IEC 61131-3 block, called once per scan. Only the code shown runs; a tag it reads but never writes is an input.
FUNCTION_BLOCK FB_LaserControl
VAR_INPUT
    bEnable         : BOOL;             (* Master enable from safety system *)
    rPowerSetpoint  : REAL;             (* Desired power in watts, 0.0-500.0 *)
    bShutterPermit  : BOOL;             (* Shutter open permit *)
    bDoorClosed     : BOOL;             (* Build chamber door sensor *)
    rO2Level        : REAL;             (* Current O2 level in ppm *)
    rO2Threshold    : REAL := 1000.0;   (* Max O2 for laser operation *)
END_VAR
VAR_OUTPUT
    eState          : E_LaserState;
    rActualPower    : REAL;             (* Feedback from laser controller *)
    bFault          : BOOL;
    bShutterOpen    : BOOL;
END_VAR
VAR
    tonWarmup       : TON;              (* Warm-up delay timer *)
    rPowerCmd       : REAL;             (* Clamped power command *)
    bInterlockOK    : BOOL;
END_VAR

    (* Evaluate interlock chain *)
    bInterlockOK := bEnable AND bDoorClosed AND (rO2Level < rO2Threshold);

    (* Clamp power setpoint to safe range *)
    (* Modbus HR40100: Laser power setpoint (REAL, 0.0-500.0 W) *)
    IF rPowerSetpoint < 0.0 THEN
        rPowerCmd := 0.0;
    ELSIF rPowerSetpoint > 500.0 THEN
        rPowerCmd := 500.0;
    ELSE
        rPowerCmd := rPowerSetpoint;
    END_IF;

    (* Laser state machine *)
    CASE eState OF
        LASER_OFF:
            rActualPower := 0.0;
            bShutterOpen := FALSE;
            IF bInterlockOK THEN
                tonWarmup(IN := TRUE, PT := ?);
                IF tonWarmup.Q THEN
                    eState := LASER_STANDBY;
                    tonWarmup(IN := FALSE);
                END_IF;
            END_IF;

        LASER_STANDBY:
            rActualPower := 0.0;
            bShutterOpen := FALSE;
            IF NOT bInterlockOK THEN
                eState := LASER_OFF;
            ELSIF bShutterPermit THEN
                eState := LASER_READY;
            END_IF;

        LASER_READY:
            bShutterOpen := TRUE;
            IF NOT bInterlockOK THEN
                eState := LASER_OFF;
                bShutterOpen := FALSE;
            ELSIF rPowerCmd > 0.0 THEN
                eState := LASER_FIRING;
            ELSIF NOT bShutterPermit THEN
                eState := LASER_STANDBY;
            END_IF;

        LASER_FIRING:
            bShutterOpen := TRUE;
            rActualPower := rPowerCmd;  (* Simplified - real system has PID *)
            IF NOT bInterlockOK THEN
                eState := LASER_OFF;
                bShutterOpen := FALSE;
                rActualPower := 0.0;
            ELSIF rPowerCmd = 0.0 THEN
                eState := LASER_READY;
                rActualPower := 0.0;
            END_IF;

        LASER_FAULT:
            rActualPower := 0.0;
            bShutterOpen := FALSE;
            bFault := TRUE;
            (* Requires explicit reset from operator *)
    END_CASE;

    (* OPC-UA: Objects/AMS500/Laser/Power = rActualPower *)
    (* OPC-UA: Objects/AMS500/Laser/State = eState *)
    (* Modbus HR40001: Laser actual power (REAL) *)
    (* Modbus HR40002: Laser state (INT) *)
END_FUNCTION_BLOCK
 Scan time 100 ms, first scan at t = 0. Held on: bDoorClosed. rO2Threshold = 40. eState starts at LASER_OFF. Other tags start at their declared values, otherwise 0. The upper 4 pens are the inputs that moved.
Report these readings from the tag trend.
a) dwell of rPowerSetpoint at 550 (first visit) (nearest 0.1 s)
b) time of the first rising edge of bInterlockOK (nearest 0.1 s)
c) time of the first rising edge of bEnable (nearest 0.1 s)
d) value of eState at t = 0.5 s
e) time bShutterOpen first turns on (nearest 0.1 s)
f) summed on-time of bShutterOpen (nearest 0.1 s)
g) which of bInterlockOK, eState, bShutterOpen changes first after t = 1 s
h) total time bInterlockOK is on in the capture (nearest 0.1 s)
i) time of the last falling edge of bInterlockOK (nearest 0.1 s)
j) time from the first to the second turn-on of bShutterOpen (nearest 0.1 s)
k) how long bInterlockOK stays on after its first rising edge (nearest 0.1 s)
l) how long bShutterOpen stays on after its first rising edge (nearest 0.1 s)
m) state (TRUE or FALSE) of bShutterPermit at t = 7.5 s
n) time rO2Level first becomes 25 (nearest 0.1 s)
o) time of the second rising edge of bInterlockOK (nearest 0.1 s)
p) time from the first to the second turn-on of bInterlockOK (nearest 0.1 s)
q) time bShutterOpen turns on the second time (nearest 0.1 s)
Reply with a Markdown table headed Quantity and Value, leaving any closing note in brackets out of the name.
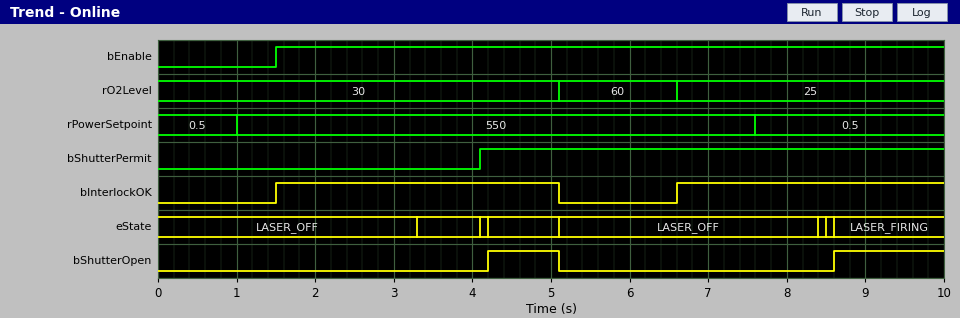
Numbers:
| Quantity | Value |
|---|---|
| dwell of rPowerSetpoint at 550 (first visit) | 6.6 s |
| time of the first rising edge of bInterlockOK | 1.5 s |
| time of the first rising edge of bEnable | 1.5 s |
| value of eState at t = 0.5 s | LASER_OFF |
| time bShutterOpen first turns on | 4.2 s |
| summed on-time of bShutterOpen | 2.3 s |
| which of bInterlockOK, eState, bShutterOpen changes first after t = 1 s | bInterlockOK |
| total time bInterlockOK is on in the capture | 7.0 s |
| time of the last falling edge of bInterlockOK | 5.1 s |
| time from the first to the second turn-on of bShutterOpen | 4.4 s |
| how long bInterlockOK stays on after its first rising edge | 3.6 s |
| how long bShutterOpen stays on after its first rising edge | 0.9 s |
| state (TRUE or FALSE) of bShutterPermit at t = 7.5 s | TRUE |
| time rO2Level first becomes 25 | 6.6 s |
| time of the second rising edge of bInterlockOK | 6.6 s |
| time from the first to the second turn-on of bInterlockOK | 5.1 s |
| time bShutterOpen turns on the second time | 8.6 s |
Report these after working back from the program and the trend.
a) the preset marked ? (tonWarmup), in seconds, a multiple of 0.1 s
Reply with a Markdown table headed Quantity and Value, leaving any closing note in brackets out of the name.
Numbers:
| Quantity | Value |
|---|---|
| the preset marked ? (tonWarmup), in seconds, a multiple of 0.1 s | 1.8 s |
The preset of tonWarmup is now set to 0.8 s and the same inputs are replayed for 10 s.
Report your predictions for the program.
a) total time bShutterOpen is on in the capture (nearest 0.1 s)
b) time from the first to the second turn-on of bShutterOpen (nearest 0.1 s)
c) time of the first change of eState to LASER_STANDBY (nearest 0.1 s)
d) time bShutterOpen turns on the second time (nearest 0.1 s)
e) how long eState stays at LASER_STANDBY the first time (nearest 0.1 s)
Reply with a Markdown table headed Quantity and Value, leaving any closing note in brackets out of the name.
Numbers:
| Quantity | Value |
|---|---|
| total time bShutterOpen is on in the capture | 3.3 s |
| time from the first to the second turn-on of bShutterOpen | 3.4 s |
| time of the first change of eState to LASER_STANDBY | 2.3 s |
| time bShutterOpen turns on the second time | 7.6 s |
| how long eState stays at LASER_STANDBY the first time | 1.8 s |
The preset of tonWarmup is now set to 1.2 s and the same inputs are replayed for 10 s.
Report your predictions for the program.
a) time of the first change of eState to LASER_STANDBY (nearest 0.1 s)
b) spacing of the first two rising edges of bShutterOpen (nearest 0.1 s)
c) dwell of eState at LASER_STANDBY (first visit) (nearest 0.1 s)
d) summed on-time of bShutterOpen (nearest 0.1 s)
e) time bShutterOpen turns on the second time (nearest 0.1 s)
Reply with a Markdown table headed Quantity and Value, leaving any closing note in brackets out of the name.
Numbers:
| Quantity | Value |
|---|---|
| time of the first change of eState to LASER_STANDBY | 2.7 s |
| spacing of the first two rising edges of bShutterOpen | 3.8 s |
| dwell of eState at LASER_STANDBY (first visit) | 1.4 s |
| summed on-time of bShutterOpen | 2.9 s |
| time bShutterOpen turns on the second time | 8.0 s |
